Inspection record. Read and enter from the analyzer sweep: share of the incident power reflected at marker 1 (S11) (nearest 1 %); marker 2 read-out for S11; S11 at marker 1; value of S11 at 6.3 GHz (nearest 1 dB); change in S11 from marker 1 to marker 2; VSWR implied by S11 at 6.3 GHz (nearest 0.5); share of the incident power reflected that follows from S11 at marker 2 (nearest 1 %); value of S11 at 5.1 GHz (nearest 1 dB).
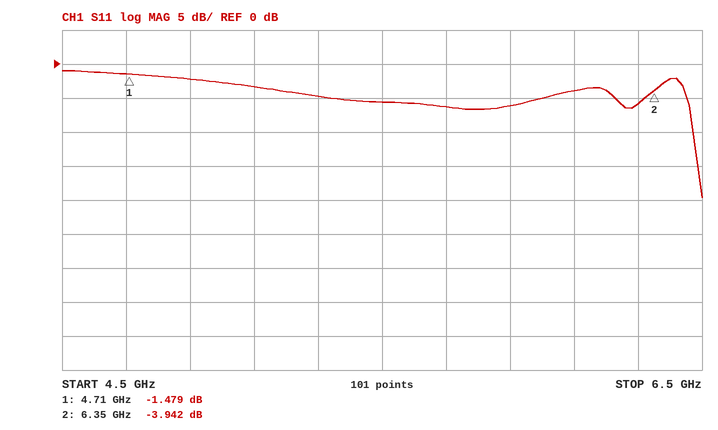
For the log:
71 %
-3.942 dB
-1.479 dB
-6 dB
-2.463 dB
3.0
40 %
-3 dB
